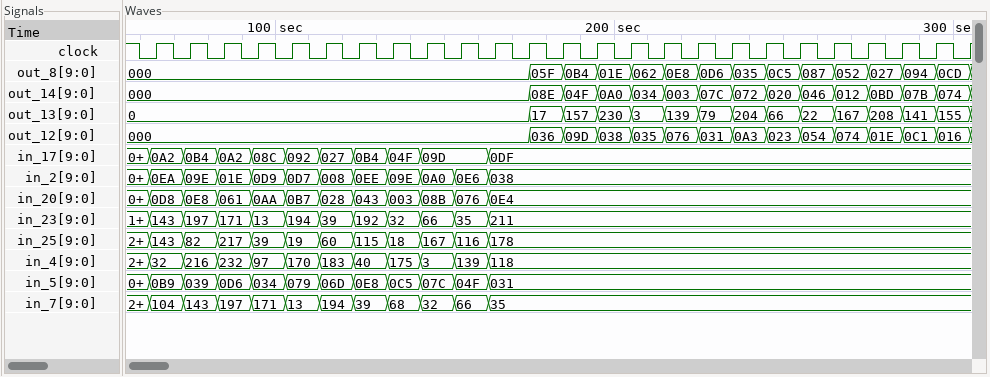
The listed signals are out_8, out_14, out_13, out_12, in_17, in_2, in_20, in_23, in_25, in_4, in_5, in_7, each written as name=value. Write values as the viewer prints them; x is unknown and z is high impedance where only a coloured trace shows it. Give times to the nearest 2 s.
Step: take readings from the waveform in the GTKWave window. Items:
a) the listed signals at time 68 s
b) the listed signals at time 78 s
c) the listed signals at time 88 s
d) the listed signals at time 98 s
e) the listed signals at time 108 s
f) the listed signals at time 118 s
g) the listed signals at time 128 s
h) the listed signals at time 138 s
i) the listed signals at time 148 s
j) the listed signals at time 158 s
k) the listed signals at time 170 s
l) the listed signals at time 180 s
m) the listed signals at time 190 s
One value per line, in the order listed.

out_8=000, out_14=000, out_13=0, out_12=000, in_17=0A2, in_2=0EA, in_20=0D8, in_23=143, in_25=143, in_4=32, in_5=0B9, in_7=104
out_8=000, out_14=000, out_13=0, out_12=000, in_17=0B4, in_2=09E, in_20=0E8, in_23=197, in_25=82, in_4=216, in_5=039, in_7=143
out_8=000, out_14=000, out_13=0, out_12=000, in_17=0A2, in_2=01E, in_20=061, in_23=171, in_25=217, in_4=232, in_5=0D6, in_7=197
out_8=000, out_14=000, out_13=0, out_12=000, in_17=08C, in_2=0D9, in_20=0AA, in_23=13, in_25=39, in_4=97, in_5=034, in_7=171
out_8=000, out_14=000, out_13=0, out_12=000, in_17=092, in_2=0D7, in_20=0B7, in_23=194, in_25=19, in_4=170, in_5=079, in_7=13
out_8=000, out_14=000, out_13=0, out_12=000, in_17=027, in_2=008, in_20=028, in_23=39, in_25=60, in_4=183, in_5=06D, in_7=194
out_8=000, out_14=000, out_13=0, out_12=000, in_17=0B4, in_2=0EE, in_20=043, in_23=192, in_25=115, in_4=40, in_5=0E8, in_7=39
out_8=000, out_14=000, out_13=0, out_12=000, in_17=04F, in_2=09E, in_20=003, in_23=32, in_25=18, in_4=175, in_5=0C5, in_7=68
out_8=000, out_14=000, out_13=0, out_12=000, in_17=09D, in_2=0A0, in_20=08B, in_23=66, in_25=167, in_4=3, in_5=07C, in_7=32
out_8=000, out_14=000, out_13=0, out_12=000, in_17=09D, in_2=0E6, in_20=076, in_23=35, in_25=116, in_4=139, in_5=04F, in_7=66
out_8=000, out_14=000, out_13=0, out_12=000, in_17=0DF, in_2=038, in_20=0E4, in_23=211, in_25=178, in_4=118, in_5=031, in_7=35
out_8=05F, out_14=08E, out_13=17, out_12=036, in_17=0DF, in_2=038, in_20=0E4, in_23=211, in_25=178, in_4=118, in_5=031, in_7=35
out_8=0B4, out_14=04F, out_13=157, out_12=09D, in_17=0DF, in_2=038, in_20=0E4, in_23=211, in_25=178, in_4=118, in_5=031, in_7=35
